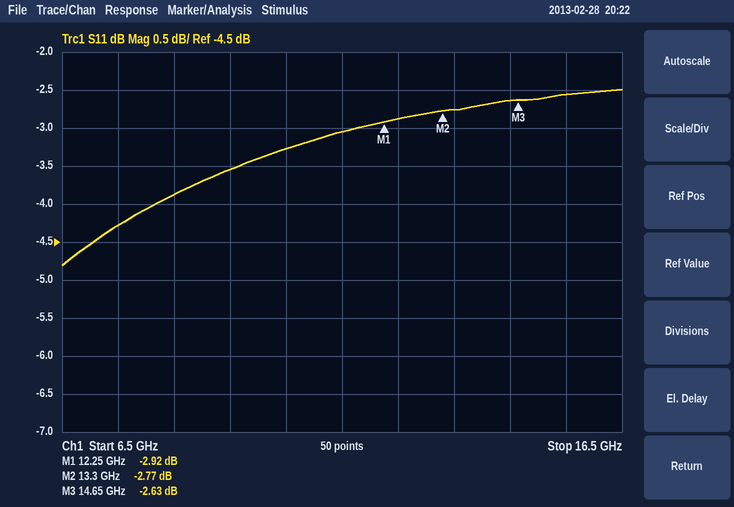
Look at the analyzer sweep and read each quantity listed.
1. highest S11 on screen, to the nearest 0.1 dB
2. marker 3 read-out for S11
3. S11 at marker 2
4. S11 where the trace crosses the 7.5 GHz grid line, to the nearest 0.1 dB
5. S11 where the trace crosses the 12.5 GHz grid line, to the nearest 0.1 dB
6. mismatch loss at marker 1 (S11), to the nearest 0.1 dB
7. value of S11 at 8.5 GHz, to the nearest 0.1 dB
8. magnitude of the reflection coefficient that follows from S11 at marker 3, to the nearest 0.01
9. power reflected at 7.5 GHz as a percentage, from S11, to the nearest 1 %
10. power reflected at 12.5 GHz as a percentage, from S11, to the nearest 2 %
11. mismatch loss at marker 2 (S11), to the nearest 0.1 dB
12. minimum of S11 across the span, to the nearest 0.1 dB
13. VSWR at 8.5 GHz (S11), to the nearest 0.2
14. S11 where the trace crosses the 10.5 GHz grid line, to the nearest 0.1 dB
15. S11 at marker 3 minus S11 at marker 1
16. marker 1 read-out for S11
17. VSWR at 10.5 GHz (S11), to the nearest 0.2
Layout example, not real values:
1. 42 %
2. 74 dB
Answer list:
1. -2.5 dB
2. -2.63 dB
3. -2.77 dB
4. -4.3 dB
5. -2.9 dB
6. 3.1 dB
7. -3.9 dB
8. 0.74
9. 37 %
10. 52 %
11. 3.3 dB
12. -4.8 dB
13. 4.6
14. -3.3 dB
15. 0.29 dB
16. -2.92 dB
17. 5.4
